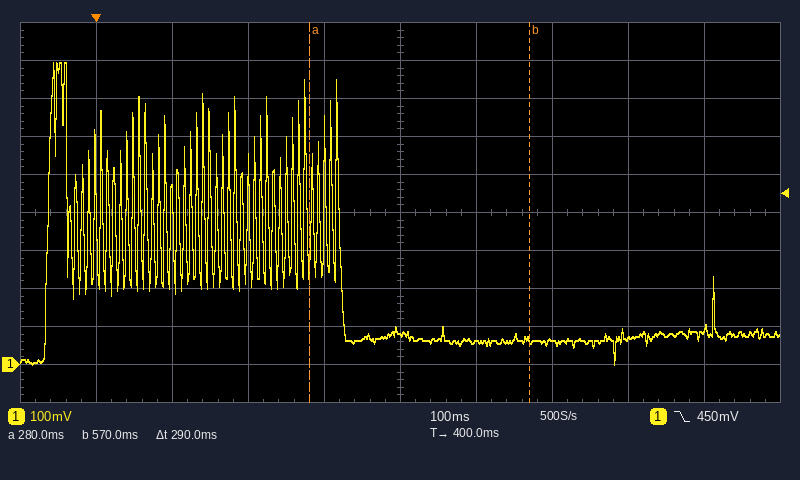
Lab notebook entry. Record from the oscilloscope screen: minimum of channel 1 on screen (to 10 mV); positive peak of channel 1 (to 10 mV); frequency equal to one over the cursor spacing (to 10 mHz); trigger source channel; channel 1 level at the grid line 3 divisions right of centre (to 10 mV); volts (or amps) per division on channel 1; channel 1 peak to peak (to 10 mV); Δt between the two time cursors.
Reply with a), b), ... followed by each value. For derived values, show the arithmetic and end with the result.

a) 0 mV
b) 790 mV
c) 1 / 290 ms ≈ 3.45 Hz
d) channel 1
e) 70 mV
f) 100 mV
g) 790 mV − (0 mV) = 790 mV
h) 290 ms
